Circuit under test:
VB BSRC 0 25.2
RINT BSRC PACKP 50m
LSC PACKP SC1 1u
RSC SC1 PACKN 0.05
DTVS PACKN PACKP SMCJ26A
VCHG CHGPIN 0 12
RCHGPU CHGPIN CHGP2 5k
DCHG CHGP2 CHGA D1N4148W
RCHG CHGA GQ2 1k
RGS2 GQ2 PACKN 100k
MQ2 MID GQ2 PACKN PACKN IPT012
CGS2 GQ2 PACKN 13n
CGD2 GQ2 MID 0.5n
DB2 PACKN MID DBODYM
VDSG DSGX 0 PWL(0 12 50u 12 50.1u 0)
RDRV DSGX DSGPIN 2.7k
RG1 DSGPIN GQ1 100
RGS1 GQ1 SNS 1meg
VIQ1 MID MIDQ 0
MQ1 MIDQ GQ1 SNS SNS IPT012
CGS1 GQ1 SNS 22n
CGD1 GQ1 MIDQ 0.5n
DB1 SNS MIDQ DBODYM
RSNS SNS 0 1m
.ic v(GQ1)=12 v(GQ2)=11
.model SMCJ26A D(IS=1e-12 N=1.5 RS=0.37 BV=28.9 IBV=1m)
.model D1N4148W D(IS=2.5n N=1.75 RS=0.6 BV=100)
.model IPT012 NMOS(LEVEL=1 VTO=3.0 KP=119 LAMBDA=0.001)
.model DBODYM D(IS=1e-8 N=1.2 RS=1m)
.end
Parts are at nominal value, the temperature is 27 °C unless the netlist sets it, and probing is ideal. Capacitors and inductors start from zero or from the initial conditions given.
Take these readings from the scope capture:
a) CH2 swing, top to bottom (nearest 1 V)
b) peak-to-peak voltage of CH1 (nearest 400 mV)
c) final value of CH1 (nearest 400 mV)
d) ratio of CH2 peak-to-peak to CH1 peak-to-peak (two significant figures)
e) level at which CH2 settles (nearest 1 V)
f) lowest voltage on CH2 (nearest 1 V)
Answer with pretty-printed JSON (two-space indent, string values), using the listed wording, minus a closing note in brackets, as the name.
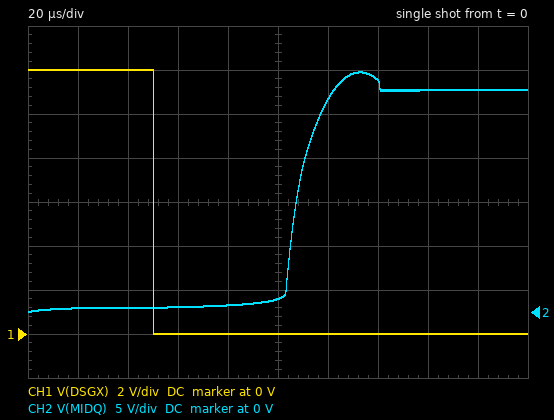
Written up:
{
  "CH2 swing, top to bottom": "27 V",
  "peak-to-peak voltage of CH1": "12.0 V",
  "final value of CH1": "0 V",
  "ratio of CH2 peak-to-peak to CH1 peak-to-peak": "2.3",
  "level at which CH2 settles": "25 V",
  "lowest voltage on CH2": "0 V"
}
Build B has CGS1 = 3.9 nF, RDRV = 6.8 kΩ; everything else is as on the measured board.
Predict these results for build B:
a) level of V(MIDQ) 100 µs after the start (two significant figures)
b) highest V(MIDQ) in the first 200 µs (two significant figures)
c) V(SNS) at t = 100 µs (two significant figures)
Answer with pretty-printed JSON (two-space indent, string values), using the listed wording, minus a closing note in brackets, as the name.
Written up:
{
  "level of V(MIDQ) 100 µs after the start": "26 V",
  "highest V(MIDQ) in the first 200 µs": "29 V",
  "V(SNS) at t = 100 µs": "59 mV"
}
